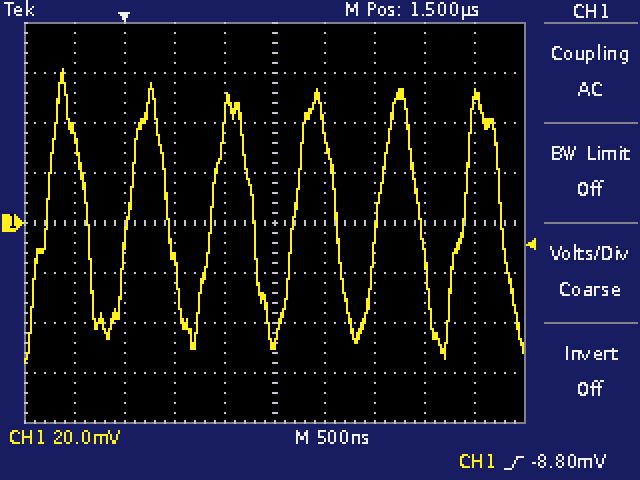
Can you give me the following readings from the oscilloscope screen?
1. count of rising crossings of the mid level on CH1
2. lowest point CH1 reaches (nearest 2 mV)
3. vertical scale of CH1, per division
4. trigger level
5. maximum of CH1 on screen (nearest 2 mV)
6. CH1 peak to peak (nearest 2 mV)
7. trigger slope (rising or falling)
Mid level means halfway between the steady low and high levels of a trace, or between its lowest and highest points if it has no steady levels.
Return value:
6
-56 mV
20 mV
-8.80 mV
62 mV
118 mV
rising
